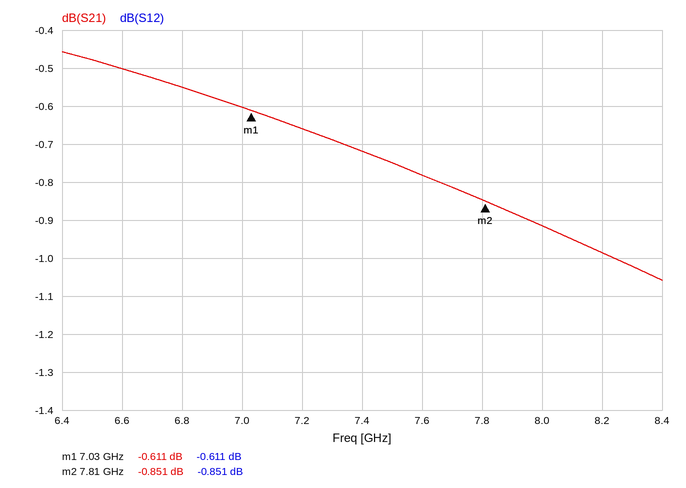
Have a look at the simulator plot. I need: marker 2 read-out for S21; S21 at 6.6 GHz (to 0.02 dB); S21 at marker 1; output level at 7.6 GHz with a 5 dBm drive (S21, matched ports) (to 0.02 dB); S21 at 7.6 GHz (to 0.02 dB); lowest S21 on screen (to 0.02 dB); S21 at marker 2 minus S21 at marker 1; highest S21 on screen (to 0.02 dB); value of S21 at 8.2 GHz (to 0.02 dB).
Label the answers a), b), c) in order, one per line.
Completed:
a) -0.851 dB
b) -0.50 dB
c) -0.611 dB
d) 4.22 dBm
e) -0.78 dB
f) -1.06 dB
g) -0.240 dB
h) -0.46 dB
i) -0.98 dB
